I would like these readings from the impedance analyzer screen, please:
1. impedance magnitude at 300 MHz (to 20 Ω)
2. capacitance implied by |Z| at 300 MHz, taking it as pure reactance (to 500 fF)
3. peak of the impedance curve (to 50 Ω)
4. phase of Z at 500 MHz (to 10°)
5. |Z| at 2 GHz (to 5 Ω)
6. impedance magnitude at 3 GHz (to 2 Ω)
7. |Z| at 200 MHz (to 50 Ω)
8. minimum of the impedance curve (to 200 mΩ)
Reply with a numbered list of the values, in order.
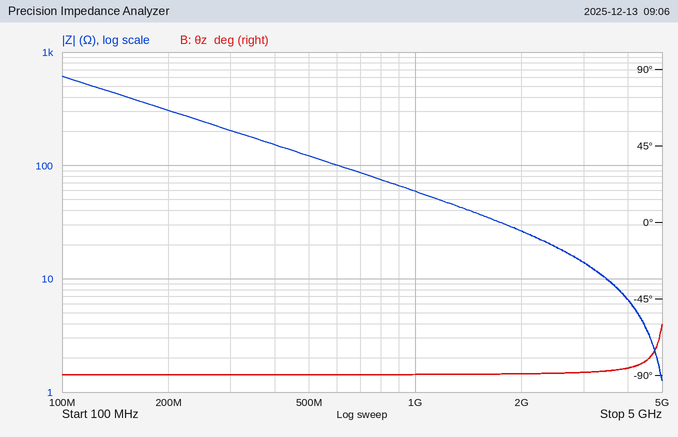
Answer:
1. 200 Ω
2. 2.5 pF
3. 600 Ω
4. -90°
5. 25 Ω
6. 14 Ω
7. 300 Ω
8. 1.2 Ω
